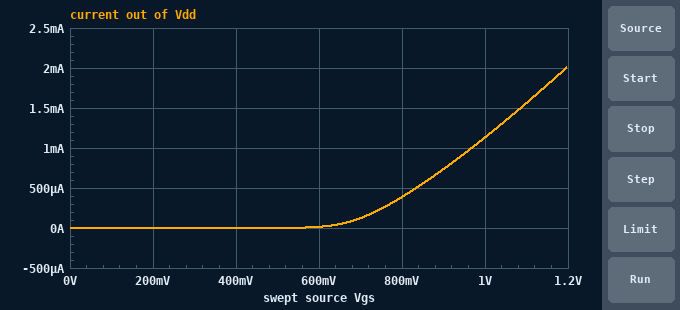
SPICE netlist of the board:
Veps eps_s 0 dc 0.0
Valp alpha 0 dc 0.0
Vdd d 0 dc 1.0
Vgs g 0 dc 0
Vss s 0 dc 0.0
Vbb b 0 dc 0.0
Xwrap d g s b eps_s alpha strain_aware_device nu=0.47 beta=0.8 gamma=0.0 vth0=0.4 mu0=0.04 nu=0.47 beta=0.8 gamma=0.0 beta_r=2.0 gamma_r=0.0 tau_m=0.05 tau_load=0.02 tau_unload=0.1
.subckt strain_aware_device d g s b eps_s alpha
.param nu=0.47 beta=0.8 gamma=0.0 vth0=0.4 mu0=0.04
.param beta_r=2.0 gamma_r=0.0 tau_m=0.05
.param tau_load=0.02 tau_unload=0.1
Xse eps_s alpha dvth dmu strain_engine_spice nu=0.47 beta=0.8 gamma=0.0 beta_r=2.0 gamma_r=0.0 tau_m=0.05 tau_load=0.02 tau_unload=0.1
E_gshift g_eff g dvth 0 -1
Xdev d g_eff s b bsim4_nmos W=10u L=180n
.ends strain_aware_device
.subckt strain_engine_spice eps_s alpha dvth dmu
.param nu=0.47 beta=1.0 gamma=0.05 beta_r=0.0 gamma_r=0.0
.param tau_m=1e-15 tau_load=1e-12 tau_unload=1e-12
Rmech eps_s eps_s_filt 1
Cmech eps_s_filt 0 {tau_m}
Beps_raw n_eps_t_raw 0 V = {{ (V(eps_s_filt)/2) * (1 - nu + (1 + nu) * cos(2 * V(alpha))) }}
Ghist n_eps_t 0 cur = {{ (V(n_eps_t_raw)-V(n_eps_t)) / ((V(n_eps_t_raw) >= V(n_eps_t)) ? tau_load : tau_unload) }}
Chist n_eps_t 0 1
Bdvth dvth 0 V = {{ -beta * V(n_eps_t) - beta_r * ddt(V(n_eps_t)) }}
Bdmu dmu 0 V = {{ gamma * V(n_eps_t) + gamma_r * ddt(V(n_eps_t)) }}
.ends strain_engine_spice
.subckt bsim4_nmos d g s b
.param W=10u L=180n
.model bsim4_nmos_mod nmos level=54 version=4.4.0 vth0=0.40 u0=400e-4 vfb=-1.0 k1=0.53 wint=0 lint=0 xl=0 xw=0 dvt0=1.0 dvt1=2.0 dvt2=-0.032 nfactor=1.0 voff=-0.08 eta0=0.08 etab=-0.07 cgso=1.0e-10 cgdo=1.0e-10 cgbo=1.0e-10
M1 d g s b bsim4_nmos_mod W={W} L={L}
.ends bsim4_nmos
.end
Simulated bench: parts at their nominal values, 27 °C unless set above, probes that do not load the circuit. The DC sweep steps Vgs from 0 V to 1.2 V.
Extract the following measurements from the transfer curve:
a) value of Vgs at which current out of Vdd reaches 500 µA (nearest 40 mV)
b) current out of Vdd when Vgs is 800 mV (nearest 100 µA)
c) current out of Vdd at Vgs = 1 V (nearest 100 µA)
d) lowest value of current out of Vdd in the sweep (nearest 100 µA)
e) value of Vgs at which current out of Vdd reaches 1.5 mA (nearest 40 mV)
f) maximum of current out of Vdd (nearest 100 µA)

840 mV
400 µA
1.1 mA
0 A
1.08 V
2.0 mA
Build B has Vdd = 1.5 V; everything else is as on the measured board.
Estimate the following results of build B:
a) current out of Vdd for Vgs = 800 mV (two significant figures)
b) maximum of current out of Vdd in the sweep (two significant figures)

440 µA
2.2 mA
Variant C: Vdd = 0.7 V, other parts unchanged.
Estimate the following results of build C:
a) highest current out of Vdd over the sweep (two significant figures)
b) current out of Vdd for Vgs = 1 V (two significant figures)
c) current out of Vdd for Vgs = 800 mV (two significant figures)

1.9 mA
1.0 mA
350 µA
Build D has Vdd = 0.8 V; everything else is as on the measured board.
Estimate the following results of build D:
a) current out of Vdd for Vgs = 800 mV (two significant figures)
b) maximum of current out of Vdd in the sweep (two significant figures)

360 µA
1.9 mA
